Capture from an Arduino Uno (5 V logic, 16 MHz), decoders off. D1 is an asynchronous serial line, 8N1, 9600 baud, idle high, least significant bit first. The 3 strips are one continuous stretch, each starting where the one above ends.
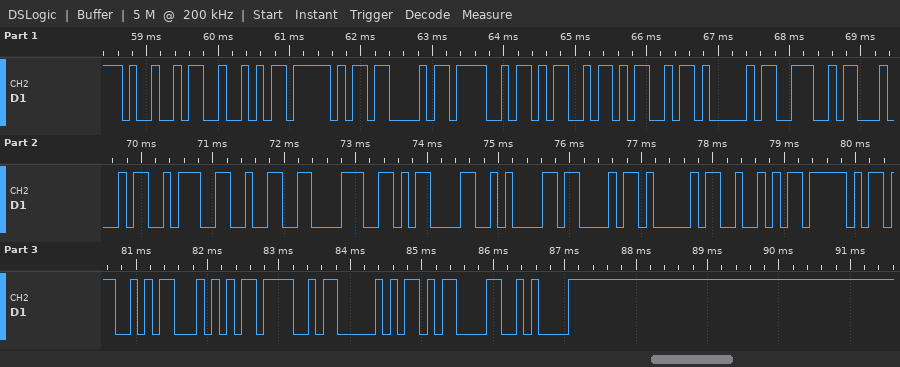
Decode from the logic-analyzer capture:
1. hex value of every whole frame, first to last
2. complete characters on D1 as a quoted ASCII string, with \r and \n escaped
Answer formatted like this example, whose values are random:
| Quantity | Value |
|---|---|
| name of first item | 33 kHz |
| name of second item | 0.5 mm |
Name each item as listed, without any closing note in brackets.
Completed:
| Quantity | Value |
|---|---|
| hex value of every whole frame, first to last | 0x49 0x52 0x5F 0x43 0x4F 0x4D 0x4D 0x41 0x4E 0x44 0x3A 0x32 0x38 0x0D 0x0A 0x43 0x41 0x52 0x5F 0x53 0x54 0x4F 0x50 0x0D 0x0A |
| complete characters on D1 as a quoted ASCII string, with \r and \n escaped | "IR_COMMAND:28\r\nCAR_STOP\r\n" |
